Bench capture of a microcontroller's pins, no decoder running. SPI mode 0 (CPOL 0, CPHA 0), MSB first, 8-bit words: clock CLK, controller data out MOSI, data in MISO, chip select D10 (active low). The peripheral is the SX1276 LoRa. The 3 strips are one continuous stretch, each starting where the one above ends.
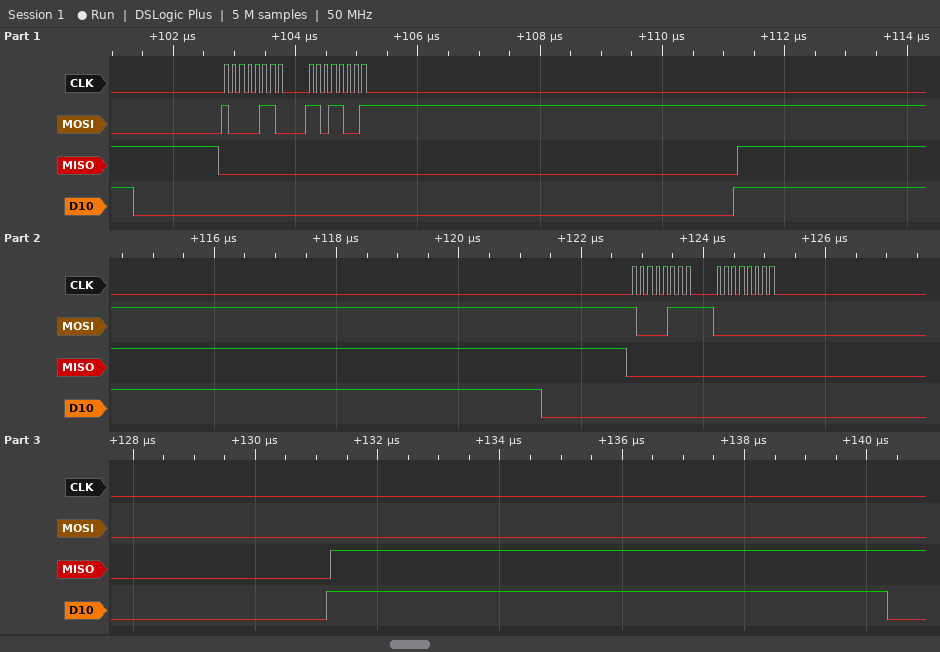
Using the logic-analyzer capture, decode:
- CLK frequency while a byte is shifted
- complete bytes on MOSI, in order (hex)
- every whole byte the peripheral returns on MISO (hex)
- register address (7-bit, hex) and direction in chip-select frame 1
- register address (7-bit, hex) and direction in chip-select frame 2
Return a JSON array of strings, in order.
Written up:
["8 MHz", "0x86 0xD9 0x87 0x00", "0x00 0x00 0x00 0x00", "0x06 write", "0x07 write"]
